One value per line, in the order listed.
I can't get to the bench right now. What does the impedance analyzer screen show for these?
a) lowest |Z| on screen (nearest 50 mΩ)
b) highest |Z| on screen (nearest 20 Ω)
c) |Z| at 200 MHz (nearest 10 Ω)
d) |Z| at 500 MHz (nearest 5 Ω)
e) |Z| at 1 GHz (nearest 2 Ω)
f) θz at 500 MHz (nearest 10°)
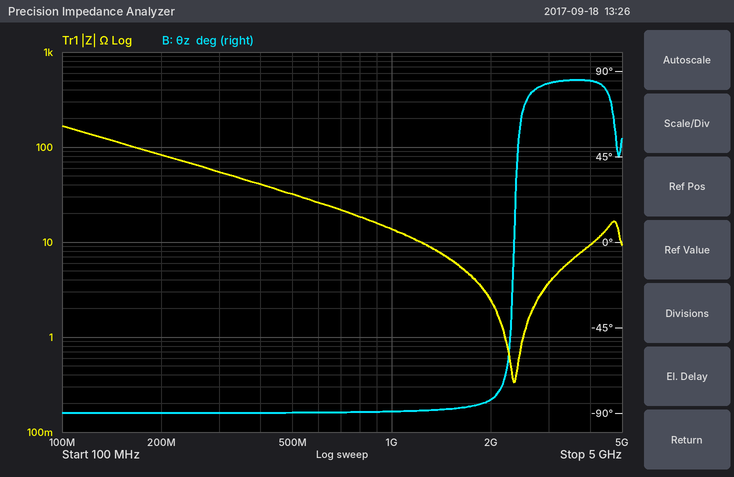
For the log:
350 mΩ
160 Ω
80 Ω
30 Ω
14 Ω
-90°
